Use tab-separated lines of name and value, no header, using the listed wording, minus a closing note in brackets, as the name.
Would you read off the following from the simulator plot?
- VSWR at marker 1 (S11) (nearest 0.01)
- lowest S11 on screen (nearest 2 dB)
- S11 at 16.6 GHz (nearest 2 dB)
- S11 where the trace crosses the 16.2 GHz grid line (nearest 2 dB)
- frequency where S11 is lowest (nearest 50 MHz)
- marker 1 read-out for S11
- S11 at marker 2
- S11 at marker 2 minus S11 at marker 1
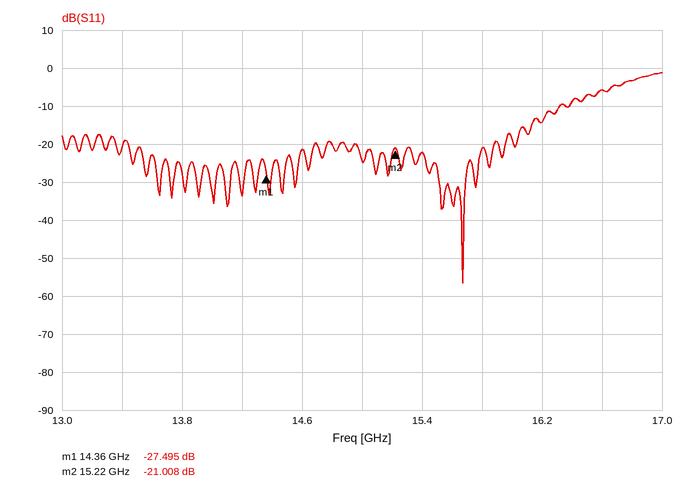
VSWR at marker 1 (S11)	1.09
lowest S11 on screen	-56 dB
S11 at 16.6 GHz	-6 dB
S11 where the trace crosses the 16.2 GHz grid line	-14 dB
frequency where S11 is lowest	15.65 GHz
marker 1 read-out for S11	-27.495 dB
S11 at marker 2	-21.008 dB
S11 at marker 2 minus S11 at marker 1	6.487 dB
